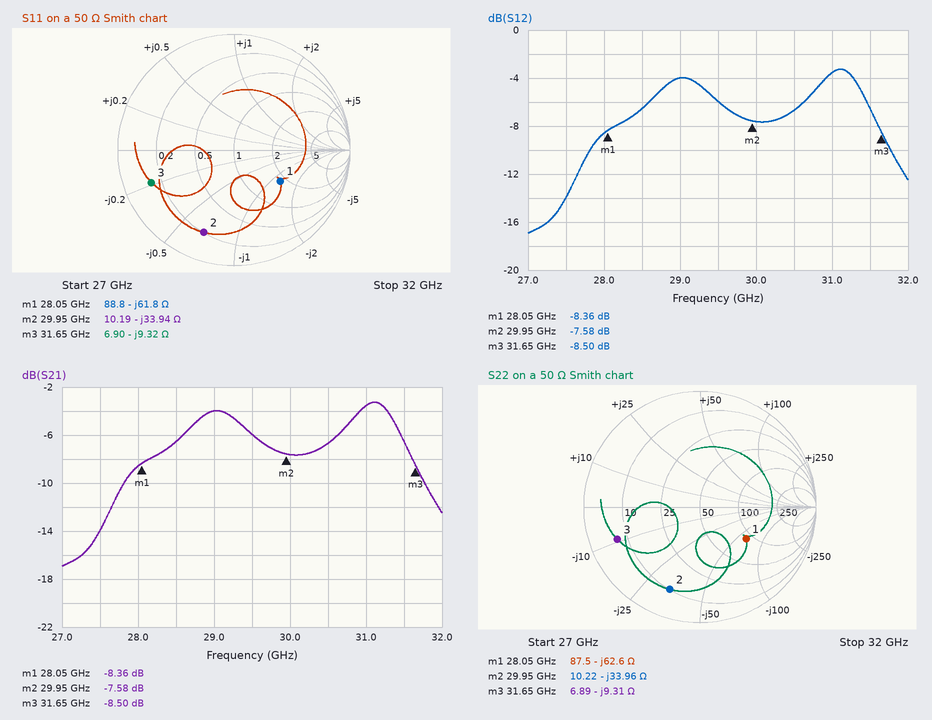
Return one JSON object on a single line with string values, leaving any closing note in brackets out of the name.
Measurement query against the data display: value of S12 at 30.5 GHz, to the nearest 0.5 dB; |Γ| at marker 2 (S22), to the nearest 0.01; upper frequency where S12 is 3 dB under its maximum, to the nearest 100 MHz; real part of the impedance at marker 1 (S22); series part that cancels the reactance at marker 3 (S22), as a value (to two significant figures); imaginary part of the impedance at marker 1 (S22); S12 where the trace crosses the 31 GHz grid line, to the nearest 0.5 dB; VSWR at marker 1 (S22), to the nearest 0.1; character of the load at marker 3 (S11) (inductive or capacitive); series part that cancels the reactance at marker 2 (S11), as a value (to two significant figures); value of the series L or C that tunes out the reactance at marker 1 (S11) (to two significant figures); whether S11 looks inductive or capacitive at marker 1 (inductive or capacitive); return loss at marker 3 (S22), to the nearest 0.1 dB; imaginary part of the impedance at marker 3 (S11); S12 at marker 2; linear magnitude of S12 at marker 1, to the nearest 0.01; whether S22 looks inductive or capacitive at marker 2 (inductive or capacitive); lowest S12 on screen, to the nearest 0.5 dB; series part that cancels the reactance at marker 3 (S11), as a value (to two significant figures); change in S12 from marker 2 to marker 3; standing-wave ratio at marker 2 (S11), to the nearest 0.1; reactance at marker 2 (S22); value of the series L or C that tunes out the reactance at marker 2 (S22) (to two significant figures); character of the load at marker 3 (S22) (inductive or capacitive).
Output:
{"value of S12 at 30.5 GHz, to the nearest 0.5 dB": "-6.5 dB", "|Γ| at marker 2 (S22), to the nearest 0.01": "0.76", "upper frequency where S12 is 3 dB under its maximum, to the nearest 100 MHz": "31.5 GHz", "real part of the impedance at marker 1": "87.5 Ω", "series part that cancels the reactance at marker 3 (S22), as a value": "47 pH", "imaginary part of the impedance at marker 1": "-62.6 Ω", "S12 where the trace crosses the 31 GHz grid line, to the nearest 0.5 dB": "-3.5 dB", "VSWR at marker 1 (S22), to the nearest 0.1": "2.9", "character of the load at marker 3 (S11)": "capacitive", "series part that cancels the reactance at marker 2 (S11), as a value": "180 pH", "value of the series L or C that tunes out the reactance at marker 1 (S11)": "350 pH", "whether S11 looks inductive or capacitive at marker 1": "capacitive", "return loss at marker 3 (S22), to the nearest 0.1 dB": "2.3 dB", "imaginary part of the impedance at marker 3": "-9.32 Ω", "S12 at marker 2": "-7.58 dB", "linear magnitude of S12 at marker 1, to the nearest 0.01": "0.38", "whether S22 looks inductive or capacitive at marker 2": "capacitive", "lowest S12 on screen, to the nearest 0.5 dB": "-17.0 dB", "series part that cancels the reactance at marker 3 (S11), as a value": "47 pH", "change in S12 from marker 2 to marker 3": "-0.92 dB", "standing-wave ratio at marker 2 (S11), to the nearest 0.1": "7.2", "reactance at marker 2": "-33.96 Ω", "value of the series L or C that tunes out the reactance at marker 2 (S22)": "180 pH", "character of the load at marker 3 (S22)": "capacitive"}
